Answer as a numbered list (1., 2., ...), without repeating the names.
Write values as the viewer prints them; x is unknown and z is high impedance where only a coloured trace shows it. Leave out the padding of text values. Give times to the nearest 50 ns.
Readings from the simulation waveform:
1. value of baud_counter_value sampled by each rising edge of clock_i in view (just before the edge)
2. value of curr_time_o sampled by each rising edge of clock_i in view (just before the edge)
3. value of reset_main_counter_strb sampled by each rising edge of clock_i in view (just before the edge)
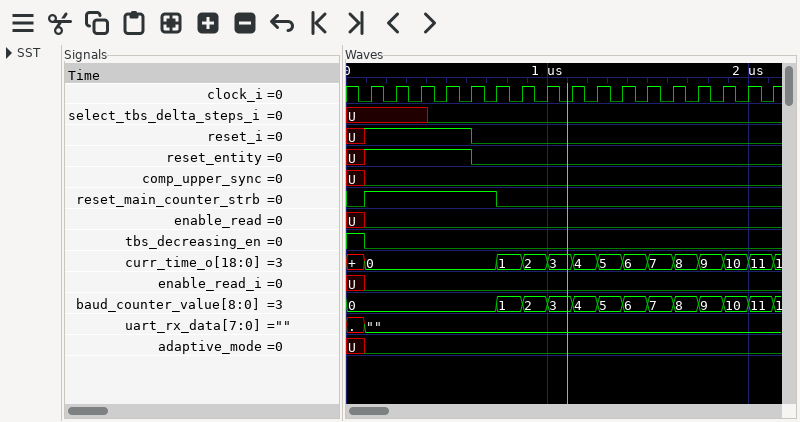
1. 0, 0, 0, 0, 0, 0, 1, 2, 3, 4, 5, 6, 7, 8, 9, 10, 11
2. 0, 0, 0, 0, 0, 0, 1, 2, 3, 4, 5, 6, 7, 8, 9, 10, 11
3. 1 1 1 1 1 1 0 0 0 0 0 0 0 0 0 0 0
